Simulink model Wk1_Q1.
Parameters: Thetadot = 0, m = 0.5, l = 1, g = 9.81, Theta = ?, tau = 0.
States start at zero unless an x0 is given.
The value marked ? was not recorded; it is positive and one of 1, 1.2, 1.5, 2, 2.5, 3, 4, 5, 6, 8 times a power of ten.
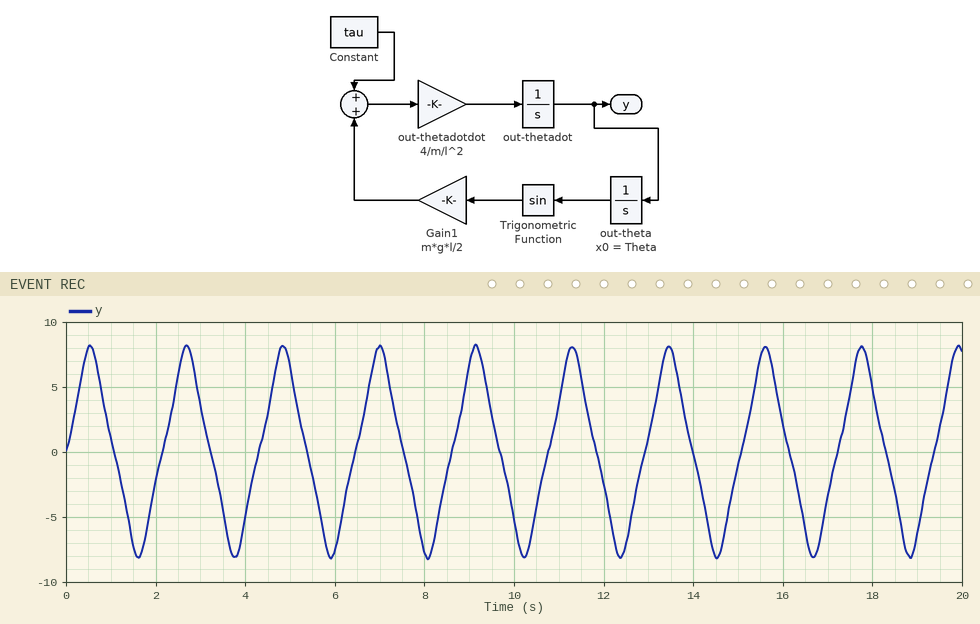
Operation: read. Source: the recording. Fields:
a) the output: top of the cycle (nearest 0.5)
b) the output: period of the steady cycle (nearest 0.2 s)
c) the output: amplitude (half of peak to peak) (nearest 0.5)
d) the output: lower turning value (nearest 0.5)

8.0
2.2 s
8.0
-8.0
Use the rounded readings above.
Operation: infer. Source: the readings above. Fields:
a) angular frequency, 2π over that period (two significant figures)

2.9 rad/s
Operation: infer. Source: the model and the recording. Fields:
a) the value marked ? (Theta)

0.8
